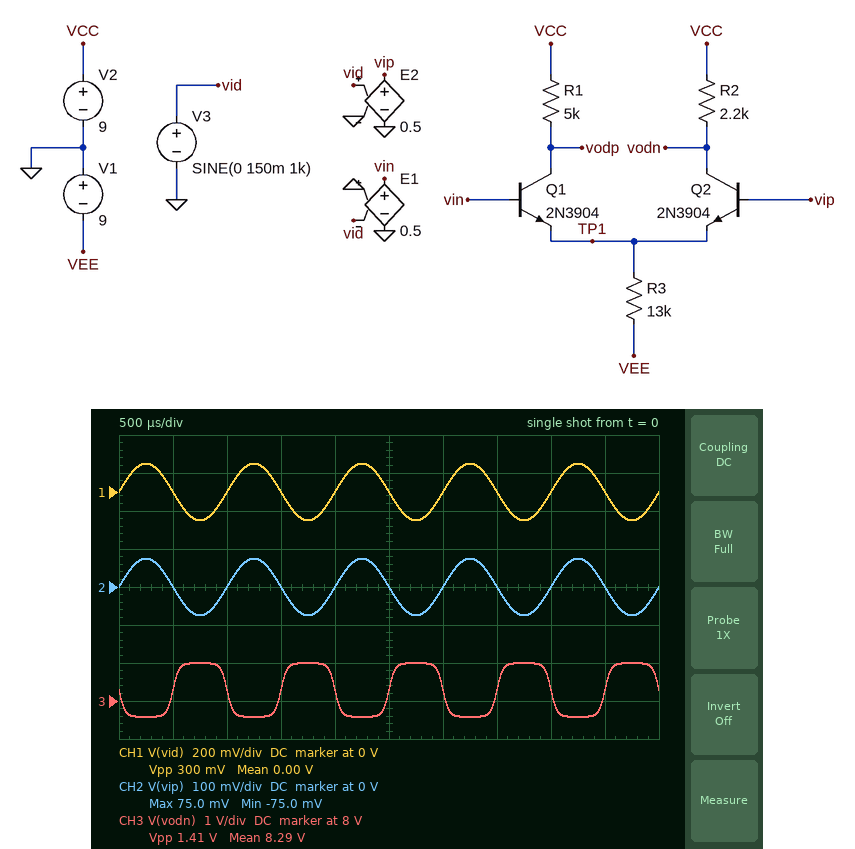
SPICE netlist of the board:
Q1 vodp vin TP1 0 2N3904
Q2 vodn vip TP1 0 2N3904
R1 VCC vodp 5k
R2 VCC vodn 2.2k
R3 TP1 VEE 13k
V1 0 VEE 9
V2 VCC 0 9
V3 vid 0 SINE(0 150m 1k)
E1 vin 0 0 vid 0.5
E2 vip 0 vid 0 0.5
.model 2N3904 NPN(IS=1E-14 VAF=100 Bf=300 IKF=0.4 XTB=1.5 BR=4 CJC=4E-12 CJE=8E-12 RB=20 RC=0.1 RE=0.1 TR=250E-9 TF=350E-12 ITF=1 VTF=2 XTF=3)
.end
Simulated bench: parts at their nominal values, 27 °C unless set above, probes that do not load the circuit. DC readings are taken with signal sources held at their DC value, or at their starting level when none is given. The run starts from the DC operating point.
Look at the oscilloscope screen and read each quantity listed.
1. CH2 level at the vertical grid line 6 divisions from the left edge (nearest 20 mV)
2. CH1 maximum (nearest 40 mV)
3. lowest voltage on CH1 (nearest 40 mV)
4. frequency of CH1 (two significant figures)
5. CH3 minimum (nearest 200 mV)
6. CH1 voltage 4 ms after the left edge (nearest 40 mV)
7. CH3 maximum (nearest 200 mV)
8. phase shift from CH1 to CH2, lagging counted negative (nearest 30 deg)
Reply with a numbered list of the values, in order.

1. 0 V
2. 160 mV
3. -160 mV
4. 1.0 kHz
5. 7.6 V
6. 0 V
7. 9.0 V
8. 0 deg
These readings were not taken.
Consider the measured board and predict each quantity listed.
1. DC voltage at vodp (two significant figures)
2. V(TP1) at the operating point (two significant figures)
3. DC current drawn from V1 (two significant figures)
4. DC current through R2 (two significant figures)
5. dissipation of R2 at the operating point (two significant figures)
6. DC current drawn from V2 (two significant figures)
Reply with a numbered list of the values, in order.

1. 7.4 V
2. -620 mV
3. 640 µA
4. 320 µA
5. 230 µW
6. 640 µA
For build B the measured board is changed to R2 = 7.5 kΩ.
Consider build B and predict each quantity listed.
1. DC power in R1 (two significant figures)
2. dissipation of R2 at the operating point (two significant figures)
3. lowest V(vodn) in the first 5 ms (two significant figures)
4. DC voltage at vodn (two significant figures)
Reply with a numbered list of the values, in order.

1. 520 µW
2. 770 µW
3. 4.2 V
4. 6.6 V
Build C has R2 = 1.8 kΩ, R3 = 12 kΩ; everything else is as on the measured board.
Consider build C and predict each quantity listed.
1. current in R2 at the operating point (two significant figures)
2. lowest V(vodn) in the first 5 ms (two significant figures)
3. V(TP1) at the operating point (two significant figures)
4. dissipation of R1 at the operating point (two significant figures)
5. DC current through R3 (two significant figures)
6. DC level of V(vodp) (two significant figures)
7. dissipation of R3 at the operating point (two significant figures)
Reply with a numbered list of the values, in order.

1. 350 µA
2. 7.7 V
3. -630 mV
4. 600 µW
5. 700 µA
6. 7.3 V
7. 5.8 mW
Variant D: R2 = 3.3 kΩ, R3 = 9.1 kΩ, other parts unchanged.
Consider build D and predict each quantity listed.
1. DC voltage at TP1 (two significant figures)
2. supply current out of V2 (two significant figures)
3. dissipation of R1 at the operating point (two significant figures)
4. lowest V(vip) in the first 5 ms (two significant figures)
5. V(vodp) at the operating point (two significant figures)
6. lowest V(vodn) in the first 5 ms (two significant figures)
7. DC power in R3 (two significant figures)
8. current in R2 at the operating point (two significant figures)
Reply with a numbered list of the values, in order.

1. -630 mV
2. 920 µA
3. 1.0 mW
4. -75 mV
5. 6.7 V
6. 6.0 V
7. 7.7 mW
8. 460 µA
